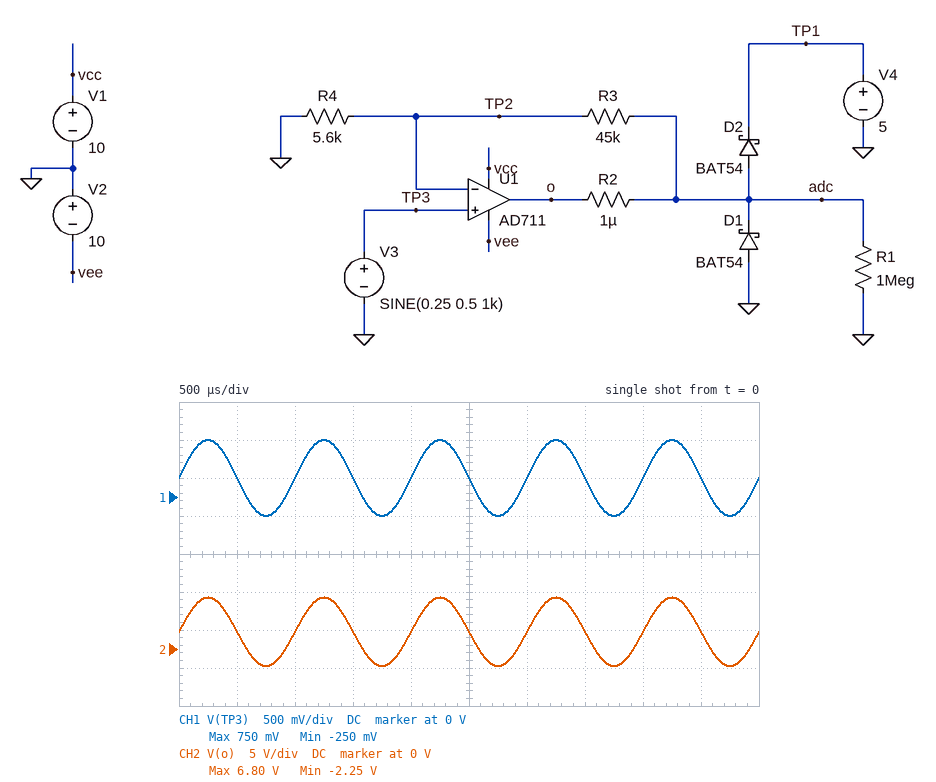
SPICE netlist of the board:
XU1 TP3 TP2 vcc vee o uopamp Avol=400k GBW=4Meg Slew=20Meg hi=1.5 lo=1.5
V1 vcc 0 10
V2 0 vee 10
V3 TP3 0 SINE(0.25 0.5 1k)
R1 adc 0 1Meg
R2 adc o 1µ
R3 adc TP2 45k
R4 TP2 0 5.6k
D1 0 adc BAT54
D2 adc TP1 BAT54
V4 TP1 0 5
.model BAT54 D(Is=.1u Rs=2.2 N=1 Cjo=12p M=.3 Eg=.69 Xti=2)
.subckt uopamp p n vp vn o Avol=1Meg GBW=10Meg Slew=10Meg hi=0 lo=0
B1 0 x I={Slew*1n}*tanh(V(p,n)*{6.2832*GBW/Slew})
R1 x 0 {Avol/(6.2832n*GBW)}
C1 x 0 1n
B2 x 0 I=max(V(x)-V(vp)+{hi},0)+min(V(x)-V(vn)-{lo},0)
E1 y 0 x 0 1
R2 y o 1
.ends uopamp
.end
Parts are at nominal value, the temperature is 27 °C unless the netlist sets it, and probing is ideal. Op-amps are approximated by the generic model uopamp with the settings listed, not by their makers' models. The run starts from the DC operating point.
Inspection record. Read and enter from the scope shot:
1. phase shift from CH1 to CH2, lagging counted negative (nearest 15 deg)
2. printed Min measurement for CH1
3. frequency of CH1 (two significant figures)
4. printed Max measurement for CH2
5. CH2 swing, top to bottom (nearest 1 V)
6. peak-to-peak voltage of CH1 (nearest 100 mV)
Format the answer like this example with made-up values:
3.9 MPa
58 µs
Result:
0 deg
-250 mV
1.0 kHz
6.80 V
9 V
1.0 V
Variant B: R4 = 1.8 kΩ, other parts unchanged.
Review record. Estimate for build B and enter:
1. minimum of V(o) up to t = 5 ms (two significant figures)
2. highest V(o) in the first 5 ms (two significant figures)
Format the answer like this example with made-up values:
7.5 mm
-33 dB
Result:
-6.0 V
7.5 V
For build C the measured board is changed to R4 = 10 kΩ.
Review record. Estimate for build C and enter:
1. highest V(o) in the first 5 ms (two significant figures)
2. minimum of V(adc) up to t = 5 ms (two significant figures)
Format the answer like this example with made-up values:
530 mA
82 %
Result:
4.1 V
-1.4 V
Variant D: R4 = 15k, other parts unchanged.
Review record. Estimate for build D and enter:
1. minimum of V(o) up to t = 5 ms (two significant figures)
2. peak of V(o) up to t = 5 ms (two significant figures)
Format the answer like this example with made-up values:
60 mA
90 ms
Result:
-1.0 V
3.0 V
